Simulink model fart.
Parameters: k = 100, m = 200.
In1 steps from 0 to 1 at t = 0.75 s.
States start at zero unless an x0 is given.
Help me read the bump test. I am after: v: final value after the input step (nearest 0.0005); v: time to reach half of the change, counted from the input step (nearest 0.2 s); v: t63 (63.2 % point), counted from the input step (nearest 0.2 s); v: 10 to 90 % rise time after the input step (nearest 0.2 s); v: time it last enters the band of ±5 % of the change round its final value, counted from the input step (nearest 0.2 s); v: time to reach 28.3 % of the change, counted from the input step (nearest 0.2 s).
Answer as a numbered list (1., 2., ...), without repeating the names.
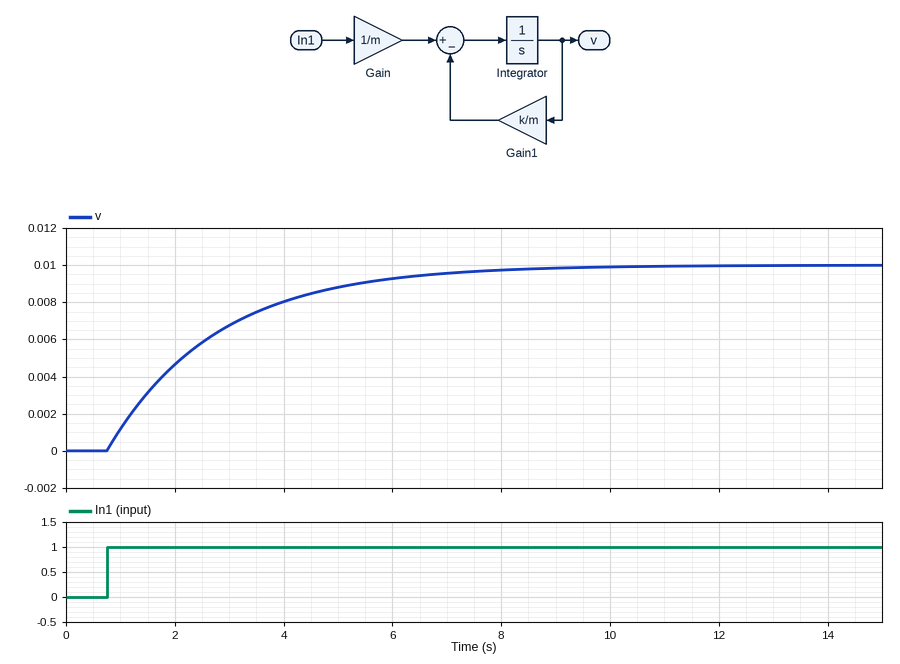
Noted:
1. 0.0100
2. 1.4 s
3. 2.0 s
4. 4.4 s
5. 6.0 s
6. 0.6 s
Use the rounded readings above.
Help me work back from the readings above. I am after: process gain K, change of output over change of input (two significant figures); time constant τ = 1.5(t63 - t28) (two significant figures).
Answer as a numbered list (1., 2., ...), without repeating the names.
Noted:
1. 0.010
2. 2.1 s
